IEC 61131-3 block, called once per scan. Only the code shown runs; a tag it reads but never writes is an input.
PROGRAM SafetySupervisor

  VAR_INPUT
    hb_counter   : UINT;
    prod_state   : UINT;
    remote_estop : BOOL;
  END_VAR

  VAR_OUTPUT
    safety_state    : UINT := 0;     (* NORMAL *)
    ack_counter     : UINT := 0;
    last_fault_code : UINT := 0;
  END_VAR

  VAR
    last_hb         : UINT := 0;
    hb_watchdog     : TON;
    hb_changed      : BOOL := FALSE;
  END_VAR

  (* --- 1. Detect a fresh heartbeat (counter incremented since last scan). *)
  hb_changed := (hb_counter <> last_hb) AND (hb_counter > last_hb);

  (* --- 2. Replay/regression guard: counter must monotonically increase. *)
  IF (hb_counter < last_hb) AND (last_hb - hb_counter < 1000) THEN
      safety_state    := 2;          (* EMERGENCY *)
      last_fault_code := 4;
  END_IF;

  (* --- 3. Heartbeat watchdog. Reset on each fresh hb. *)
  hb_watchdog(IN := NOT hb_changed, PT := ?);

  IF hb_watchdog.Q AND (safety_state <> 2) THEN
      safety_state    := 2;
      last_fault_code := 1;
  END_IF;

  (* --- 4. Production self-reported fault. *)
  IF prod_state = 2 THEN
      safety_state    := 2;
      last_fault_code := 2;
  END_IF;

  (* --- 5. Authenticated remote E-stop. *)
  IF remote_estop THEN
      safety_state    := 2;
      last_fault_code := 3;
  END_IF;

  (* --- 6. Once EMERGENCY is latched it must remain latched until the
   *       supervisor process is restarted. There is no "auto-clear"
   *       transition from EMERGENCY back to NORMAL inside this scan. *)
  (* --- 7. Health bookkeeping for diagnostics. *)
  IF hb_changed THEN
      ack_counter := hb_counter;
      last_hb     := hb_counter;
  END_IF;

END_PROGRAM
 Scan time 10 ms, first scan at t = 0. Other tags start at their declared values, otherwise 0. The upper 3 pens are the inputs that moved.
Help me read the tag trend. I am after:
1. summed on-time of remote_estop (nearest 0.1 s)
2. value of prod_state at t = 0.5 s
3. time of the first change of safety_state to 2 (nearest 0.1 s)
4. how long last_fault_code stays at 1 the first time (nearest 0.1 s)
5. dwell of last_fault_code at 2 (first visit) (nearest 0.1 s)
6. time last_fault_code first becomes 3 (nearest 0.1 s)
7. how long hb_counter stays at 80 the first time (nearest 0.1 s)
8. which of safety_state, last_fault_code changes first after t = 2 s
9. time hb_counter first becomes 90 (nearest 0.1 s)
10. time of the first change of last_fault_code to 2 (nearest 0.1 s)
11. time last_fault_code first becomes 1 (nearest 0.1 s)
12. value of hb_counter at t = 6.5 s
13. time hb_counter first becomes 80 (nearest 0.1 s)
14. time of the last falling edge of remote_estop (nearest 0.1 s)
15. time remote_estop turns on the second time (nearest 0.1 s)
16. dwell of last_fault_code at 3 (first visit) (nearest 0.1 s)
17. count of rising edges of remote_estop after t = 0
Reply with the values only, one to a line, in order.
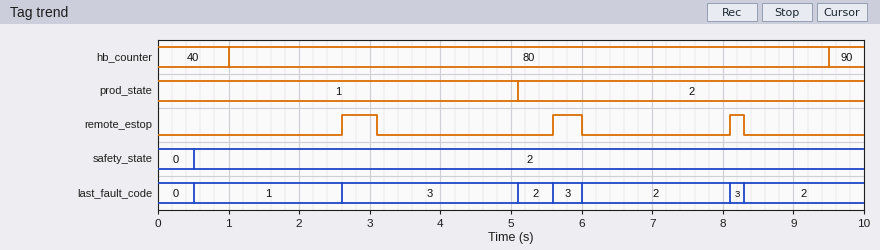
1.1 s
1
0.5 s
2.1 s
0.5 s
2.6 s
8.5 s
last_fault_code
9.5 s
5.1 s
0.5 s
80
1.0 s
8.3 s
5.6 s
2.5 s
3
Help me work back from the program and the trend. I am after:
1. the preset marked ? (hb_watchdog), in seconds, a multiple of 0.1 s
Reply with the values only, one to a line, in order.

0.5 s
